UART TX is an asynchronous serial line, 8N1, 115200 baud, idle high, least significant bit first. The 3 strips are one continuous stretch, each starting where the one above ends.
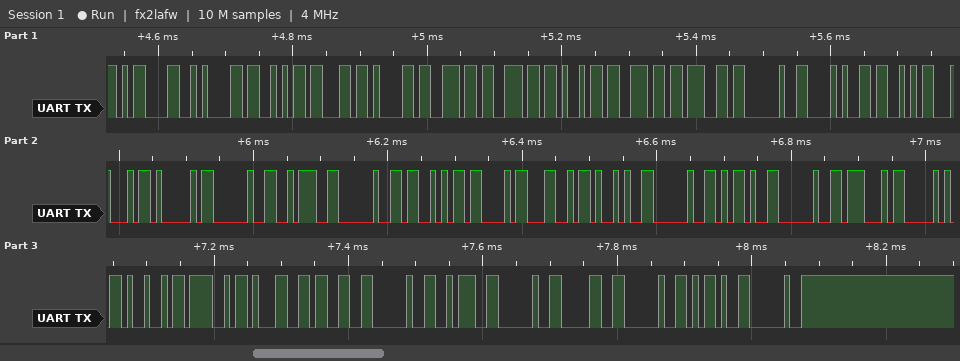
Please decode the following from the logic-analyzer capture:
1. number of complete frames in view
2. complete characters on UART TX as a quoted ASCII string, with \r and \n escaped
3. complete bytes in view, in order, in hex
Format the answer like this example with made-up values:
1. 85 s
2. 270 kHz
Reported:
1. 38
2. "\r\nScanning (SDA : SCL) - GPIO13 : 0 - "
3. 0x0D 0x0A 0x53 0x63 0x61 0x6E 0x6E 0x69 0x6E 0x67 0x20 0x28 0x53 0x44 0x41 0x20 0x3A 0x20 0x53 0x43 0x4C 0x29 0x20 0x2D 0x20 0x47 0x50 0x49 0x4F 0x31 0x33 0x20 0x3A 0x20 0x30 0x20 0x2D 0x20
